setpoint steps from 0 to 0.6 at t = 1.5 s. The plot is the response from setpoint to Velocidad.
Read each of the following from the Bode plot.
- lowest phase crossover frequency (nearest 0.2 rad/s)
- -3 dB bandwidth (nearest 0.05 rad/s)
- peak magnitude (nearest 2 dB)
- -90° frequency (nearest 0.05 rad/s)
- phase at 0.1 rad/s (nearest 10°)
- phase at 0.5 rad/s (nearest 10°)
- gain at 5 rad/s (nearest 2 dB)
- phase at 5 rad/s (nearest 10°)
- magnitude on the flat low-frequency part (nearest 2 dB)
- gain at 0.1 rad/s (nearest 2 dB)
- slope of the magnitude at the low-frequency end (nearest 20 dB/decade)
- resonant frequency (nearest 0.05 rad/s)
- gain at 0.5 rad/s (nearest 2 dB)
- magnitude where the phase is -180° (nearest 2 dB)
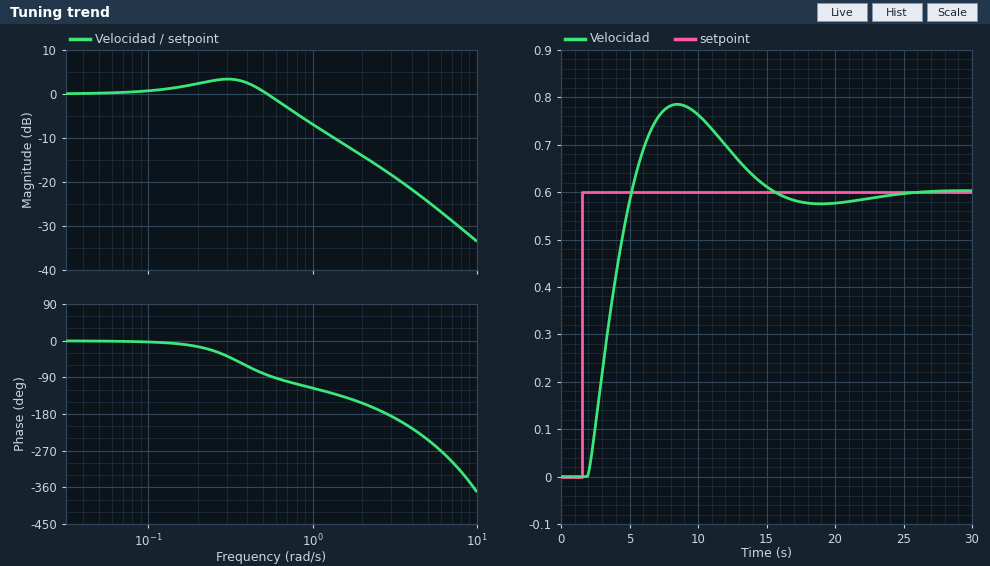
2.8 rad/s
0.70 rad/s
4 dB
0.60 rad/s
0°
-80°
-24 dB
-240°
0 dB
0 dB
0 dB/decade
0.30 rad/s
0 dB
-18 dB
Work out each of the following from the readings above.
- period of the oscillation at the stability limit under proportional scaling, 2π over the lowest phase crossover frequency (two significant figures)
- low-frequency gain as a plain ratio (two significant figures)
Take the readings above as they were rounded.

2.2 s
1.0
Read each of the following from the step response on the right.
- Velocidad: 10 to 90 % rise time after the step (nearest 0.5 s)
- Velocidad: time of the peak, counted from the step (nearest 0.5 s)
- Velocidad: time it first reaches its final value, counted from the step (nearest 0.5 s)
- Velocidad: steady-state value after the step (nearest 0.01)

2.5 s
7.0 s
3.5 s
0.60
